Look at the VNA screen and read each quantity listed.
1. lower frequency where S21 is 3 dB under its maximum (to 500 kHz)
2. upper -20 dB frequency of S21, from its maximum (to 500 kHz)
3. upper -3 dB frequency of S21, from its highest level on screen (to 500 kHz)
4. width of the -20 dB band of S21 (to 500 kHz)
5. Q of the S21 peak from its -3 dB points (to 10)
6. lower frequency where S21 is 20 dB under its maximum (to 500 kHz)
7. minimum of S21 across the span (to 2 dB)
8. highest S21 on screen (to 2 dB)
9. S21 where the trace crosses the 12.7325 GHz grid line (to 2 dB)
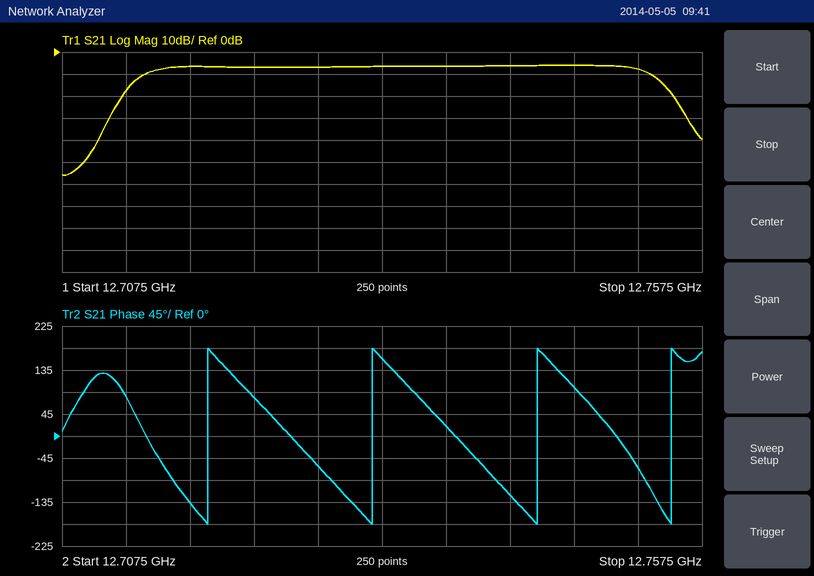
12.7145 GHz
12.7560 GHz
12.7530 GHz
44.5 MHz
330
12.7115 GHz
-56 dB
-6 dB
-6 dB
